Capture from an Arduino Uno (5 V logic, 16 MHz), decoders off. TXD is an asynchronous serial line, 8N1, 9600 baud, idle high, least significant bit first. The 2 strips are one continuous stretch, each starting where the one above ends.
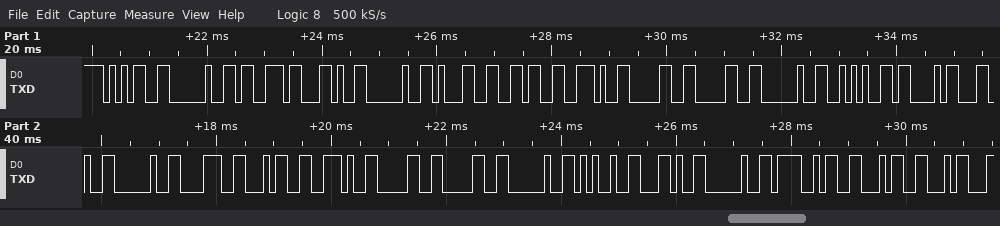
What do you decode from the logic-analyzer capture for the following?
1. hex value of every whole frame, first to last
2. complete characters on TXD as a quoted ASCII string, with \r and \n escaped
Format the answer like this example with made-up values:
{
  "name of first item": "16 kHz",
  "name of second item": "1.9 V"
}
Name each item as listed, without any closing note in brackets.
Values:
{
  "hex value of every whole frame, first to last": "0x35 0x20 0x73 0x2C 0x20 0x31 0x36 0x2E 0x30 0x30 0x20 0x2A 0x43 0x2C 0x20 0x38 0x34 0x2E 0x30 0x30 0x20 0x25 0x2C 0x20 0x4F 0x46 0x46",
  "complete characters on TXD as a quoted ASCII string, with \\r and \\n escaped": "\"5 s, 16.00 *C, 84.00 %, OFF\""
}
